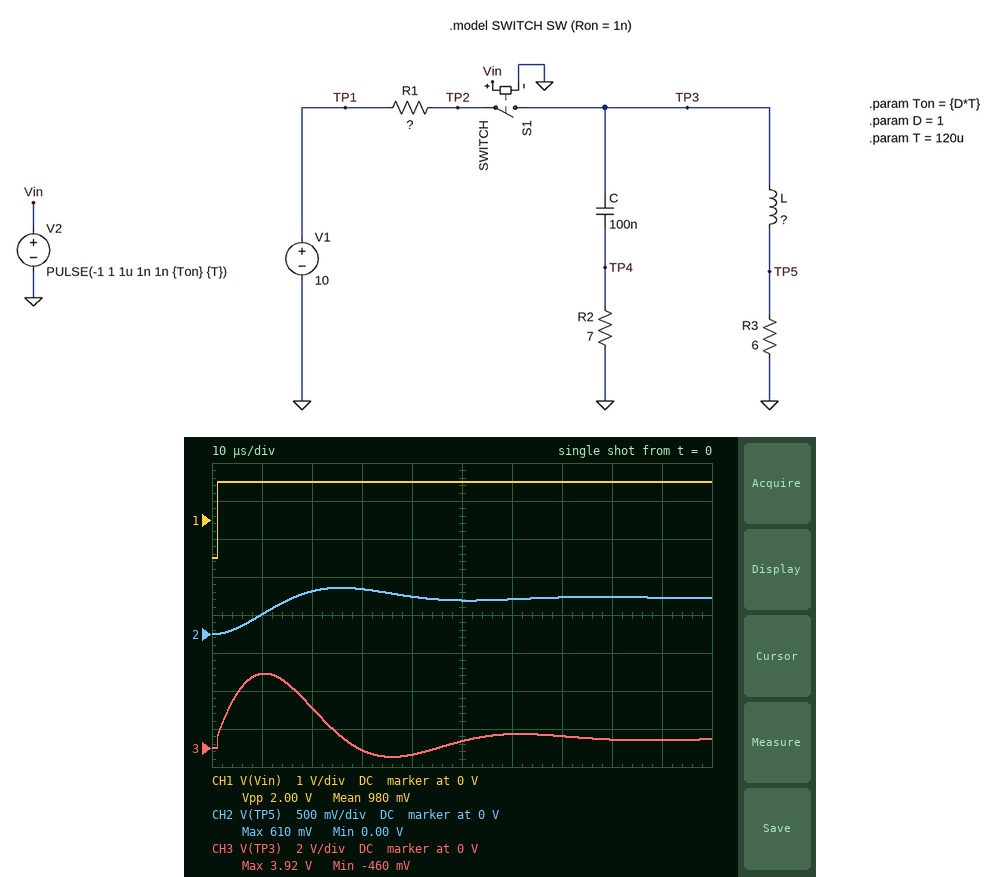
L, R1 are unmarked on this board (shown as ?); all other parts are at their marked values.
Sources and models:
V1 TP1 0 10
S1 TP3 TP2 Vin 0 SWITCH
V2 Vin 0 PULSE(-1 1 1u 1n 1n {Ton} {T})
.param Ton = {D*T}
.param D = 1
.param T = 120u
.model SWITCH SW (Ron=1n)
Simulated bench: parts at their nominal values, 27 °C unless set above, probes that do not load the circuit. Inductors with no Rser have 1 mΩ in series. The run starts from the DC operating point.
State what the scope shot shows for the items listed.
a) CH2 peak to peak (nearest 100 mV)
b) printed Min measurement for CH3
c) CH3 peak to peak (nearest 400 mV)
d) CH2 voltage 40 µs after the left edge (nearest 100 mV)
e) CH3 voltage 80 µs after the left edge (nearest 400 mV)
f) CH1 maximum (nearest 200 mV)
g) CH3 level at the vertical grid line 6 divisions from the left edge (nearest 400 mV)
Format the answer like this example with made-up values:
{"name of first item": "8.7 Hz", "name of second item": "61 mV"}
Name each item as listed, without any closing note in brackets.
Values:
{"CH2 peak to peak": "600 mV", "printed Min measurement for CH3": "-460 mV", "CH3 peak to peak": "4.4 V", "CH2 voltage 40 µs after the left edge": "500 mV", "CH3 voltage 80 µs after the left edge": "400 mV", "CH1 maximum": "1.0 V", "CH3 level at the vertical grid line 6 divisions from the left edge": "800 mV"}
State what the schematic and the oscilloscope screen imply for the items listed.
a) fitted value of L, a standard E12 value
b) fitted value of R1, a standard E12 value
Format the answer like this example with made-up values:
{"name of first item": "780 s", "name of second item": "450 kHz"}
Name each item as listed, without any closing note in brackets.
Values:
{"fitted value of L, a standard E12 value": "560 µH", "fitted value of R1, a standard E12 value": "120 Ω"}
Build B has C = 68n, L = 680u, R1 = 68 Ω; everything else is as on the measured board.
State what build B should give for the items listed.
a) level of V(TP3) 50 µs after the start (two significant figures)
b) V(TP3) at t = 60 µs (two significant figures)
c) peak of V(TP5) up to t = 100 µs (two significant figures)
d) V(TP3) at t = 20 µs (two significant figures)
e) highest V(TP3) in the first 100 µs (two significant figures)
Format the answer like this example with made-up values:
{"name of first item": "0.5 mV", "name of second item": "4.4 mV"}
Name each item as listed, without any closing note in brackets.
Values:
{"level of V(TP3) 50 µs after the start": "720 mV", "V(TP3) at t = 60 µs": "800 mV", "peak of V(TP5) up to t = 100 µs": "840 mV", "V(TP3) at t = 20 µs": "3.0 V", "highest V(TP3) in the first 100 µs": "6.3 V"}
